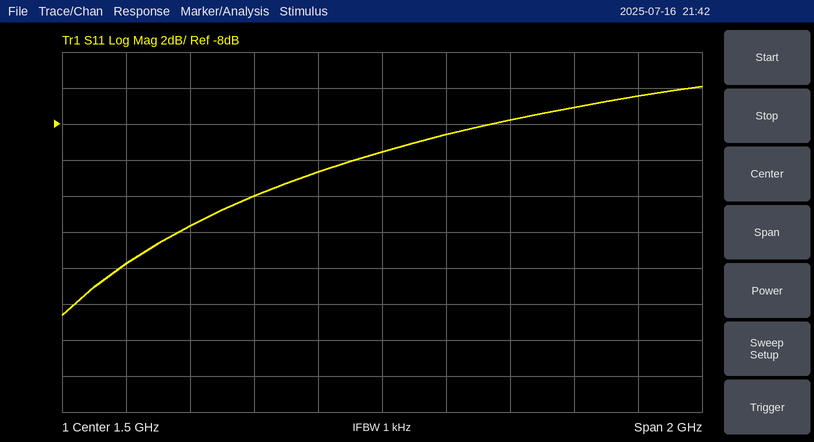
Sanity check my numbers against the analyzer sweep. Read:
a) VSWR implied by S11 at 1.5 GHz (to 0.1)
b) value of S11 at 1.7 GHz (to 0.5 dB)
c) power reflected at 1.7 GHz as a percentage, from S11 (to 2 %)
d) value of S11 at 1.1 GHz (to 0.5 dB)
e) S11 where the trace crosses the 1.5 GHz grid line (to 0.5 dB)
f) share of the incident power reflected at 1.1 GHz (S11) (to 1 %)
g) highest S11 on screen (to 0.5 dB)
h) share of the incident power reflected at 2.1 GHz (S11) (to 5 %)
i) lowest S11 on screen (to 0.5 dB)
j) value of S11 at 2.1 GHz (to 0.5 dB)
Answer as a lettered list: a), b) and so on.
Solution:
a) 2.0
b) -8.5 dB
c) 14 %
d) -12.0 dB
e) -9.5 dB
f) 6 %
g) -6.0 dB
h) 20 %
i) -18.5 dB
j) -7.0 dB
